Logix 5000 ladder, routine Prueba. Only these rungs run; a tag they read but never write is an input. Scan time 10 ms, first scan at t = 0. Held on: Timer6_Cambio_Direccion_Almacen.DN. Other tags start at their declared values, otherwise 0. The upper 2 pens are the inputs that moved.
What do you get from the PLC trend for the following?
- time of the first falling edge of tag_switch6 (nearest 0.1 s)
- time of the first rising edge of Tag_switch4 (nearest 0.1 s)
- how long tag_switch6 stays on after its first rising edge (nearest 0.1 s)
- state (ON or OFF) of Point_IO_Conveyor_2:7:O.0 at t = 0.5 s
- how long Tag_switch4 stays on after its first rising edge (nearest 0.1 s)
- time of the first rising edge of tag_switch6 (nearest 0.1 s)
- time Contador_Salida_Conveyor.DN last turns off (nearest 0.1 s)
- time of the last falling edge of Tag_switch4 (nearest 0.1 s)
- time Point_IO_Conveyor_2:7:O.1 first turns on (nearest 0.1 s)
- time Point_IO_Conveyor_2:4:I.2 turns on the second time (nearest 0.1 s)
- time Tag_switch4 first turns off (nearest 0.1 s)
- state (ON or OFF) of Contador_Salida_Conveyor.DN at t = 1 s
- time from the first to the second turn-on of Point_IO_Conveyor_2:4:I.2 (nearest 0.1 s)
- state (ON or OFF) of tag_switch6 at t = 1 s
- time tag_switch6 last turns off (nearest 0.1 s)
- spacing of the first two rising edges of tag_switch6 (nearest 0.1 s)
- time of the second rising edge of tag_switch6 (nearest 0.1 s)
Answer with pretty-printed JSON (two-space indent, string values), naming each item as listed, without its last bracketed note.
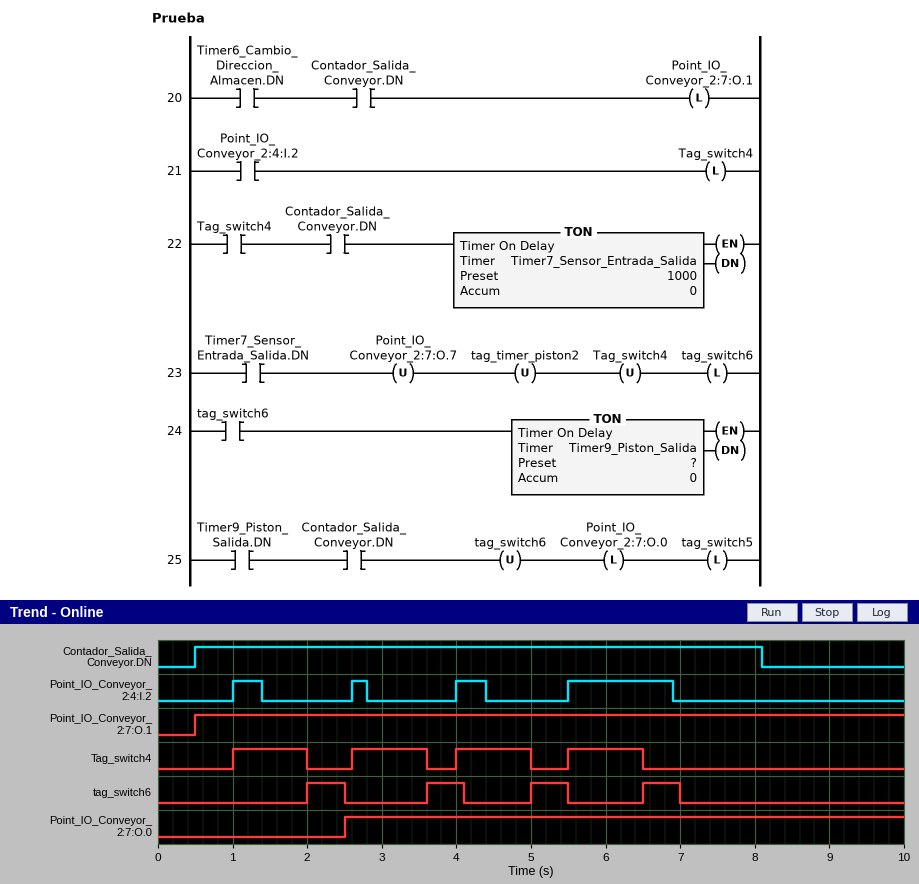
{
  "time of the first falling edge of tag_switch6": "2.5 s",
  "time of the first rising edge of Tag_switch4": "1.0 s",
  "how long tag_switch6 stays on after its first rising edge": "0.5 s",
  "state (ON or OFF) of Point_IO_Conveyor_2:7:O.0 at t = 0.5 s": "OFF",
  "how long Tag_switch4 stays on after its first rising edge": "1.0 s",
  "time of the first rising edge of tag_switch6": "2.0 s",
  "time Contador_Salida_Conveyor.DN last turns off": "8.1 s",
  "time of the last falling edge of Tag_switch4": "6.5 s",
  "time Point_IO_Conveyor_2:7:O.1 first turns on": "0.5 s",
  "time Point_IO_Conveyor_2:4:I.2 turns on the second time": "2.6 s",
  "time Tag_switch4 first turns off": "2.0 s",
  "state (ON or OFF) of Contador_Salida_Conveyor.DN at t = 1 s": "ON",
  "time from the first to the second turn-on of Point_IO_Conveyor_2:4:I.2": "1.6 s",
  "state (ON or OFF) of tag_switch6 at t = 1 s": "OFF",
  "time tag_switch6 last turns off": "7.0 s",
  "spacing of the first two rising edges of tag_switch6": "1.6 s",
  "time of the second rising edge of tag_switch6": "3.6 s"
}
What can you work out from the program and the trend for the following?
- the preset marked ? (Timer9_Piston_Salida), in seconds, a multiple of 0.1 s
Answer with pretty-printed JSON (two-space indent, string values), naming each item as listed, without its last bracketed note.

{
  "the preset marked ? (Timer9_Piston_Salida), in seconds, a multiple of 0.1 s": "0.5 s"
}
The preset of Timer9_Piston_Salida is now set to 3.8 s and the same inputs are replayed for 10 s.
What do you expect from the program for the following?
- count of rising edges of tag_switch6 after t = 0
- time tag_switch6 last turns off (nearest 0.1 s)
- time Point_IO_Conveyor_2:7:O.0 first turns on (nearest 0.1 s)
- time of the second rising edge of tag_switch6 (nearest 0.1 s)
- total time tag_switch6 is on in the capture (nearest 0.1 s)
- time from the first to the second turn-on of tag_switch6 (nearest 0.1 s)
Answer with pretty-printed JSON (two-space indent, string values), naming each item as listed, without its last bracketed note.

{
  "count of rising edges of tag_switch6 after t = 0": "2",
  "time tag_switch6 last turns off": "5.8 s",
  "time Point_IO_Conveyor_2:7:O.0 first turns on": "5.8 s",
  "time of the second rising edge of tag_switch6": "6.5 s",
  "total time tag_switch6 is on in the capture": "7.3 s",
  "time from the first to the second turn-on of tag_switch6": "4.5 s"
}
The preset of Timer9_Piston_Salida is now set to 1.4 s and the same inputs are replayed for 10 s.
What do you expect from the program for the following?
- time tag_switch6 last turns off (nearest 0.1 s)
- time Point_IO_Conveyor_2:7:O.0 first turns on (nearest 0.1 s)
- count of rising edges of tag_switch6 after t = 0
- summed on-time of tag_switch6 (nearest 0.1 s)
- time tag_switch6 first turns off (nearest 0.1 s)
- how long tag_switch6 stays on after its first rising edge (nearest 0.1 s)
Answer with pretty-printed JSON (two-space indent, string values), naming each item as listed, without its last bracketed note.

{
  "time tag_switch6 last turns off": "7.9 s",
  "time Point_IO_Conveyor_2:7:O.0 first turns on": "3.4 s",
  "count of rising edges of tag_switch6 after t = 0": "3",
  "summed on-time of tag_switch6": "4.2 s",
  "time tag_switch6 first turns off": "3.4 s",
  "how long tag_switch6 stays on after its first rising edge": "1.4 s"
}
